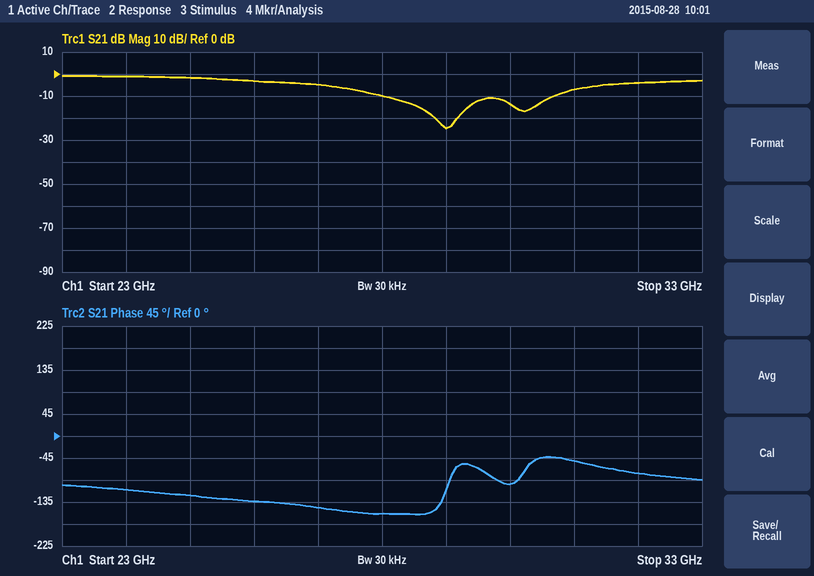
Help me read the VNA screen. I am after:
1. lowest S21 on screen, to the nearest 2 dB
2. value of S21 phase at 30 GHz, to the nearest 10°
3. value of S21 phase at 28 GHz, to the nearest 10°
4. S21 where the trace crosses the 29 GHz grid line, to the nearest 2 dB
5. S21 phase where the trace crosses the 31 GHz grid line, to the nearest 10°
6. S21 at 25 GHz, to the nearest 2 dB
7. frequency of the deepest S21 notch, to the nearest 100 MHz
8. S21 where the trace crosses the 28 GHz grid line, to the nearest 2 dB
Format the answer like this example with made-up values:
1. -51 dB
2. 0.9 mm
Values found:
1. -24 dB
2. -100°
3. -160°
4. -24 dB
5. -50°
6. -2 dB
7. 29.0 GHz
8. -10 dB
